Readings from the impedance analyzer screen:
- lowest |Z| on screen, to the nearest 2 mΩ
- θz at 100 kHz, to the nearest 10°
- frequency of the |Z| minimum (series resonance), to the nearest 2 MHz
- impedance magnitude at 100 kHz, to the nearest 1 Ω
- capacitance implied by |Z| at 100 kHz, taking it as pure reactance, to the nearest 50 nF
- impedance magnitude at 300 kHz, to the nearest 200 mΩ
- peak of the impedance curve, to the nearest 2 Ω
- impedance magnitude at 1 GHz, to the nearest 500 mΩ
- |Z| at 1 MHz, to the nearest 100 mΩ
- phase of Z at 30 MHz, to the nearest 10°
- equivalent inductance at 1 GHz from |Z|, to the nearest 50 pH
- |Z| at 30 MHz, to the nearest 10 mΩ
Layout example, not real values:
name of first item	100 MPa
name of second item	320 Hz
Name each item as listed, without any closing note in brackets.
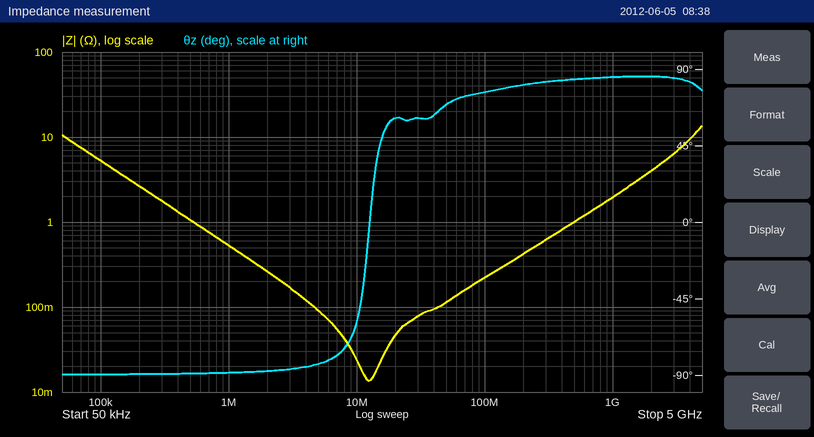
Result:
lowest |Z| on screen, to the nearest 2 mΩ	14 mΩ
θz at 100 kHz, to the nearest 10°	-90°
frequency of the |Z| minimum (series resonance), to the nearest 2 MHz	12 MHz
impedance magnitude at 100 kHz, to the nearest 1 Ω	5 Ω
capacitance implied by |Z| at 100 kHz, taking it as pure reactance, to the nearest 50 nF	300 nF
impedance magnitude at 300 kHz, to the nearest 200 mΩ	1.8 Ω
peak of the impedance curve, to the nearest 2 Ω	14 Ω
impedance magnitude at 1 GHz, to the nearest 500 mΩ	2.0 Ω
|Z| at 1 MHz, to the nearest 100 mΩ	500 mΩ
phase of Z at 30 MHz, to the nearest 10°	60°
equivalent inductance at 1 GHz from |Z|, to the nearest 50 pH	300 pH
|Z| at 30 MHz, to the nearest 10 mΩ	80 mΩ
